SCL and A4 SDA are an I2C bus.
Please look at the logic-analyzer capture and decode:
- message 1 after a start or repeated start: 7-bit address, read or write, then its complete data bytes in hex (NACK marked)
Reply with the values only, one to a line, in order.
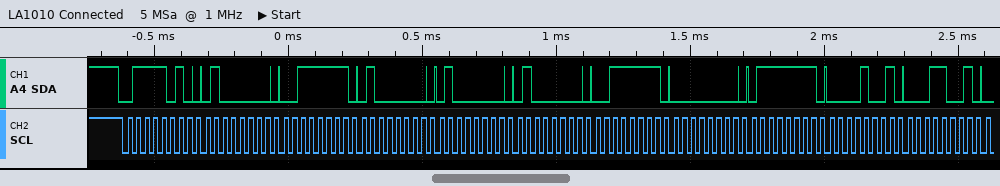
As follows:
0x3D write: 40 3F 40 40 40 3F 00 7F 09 19
